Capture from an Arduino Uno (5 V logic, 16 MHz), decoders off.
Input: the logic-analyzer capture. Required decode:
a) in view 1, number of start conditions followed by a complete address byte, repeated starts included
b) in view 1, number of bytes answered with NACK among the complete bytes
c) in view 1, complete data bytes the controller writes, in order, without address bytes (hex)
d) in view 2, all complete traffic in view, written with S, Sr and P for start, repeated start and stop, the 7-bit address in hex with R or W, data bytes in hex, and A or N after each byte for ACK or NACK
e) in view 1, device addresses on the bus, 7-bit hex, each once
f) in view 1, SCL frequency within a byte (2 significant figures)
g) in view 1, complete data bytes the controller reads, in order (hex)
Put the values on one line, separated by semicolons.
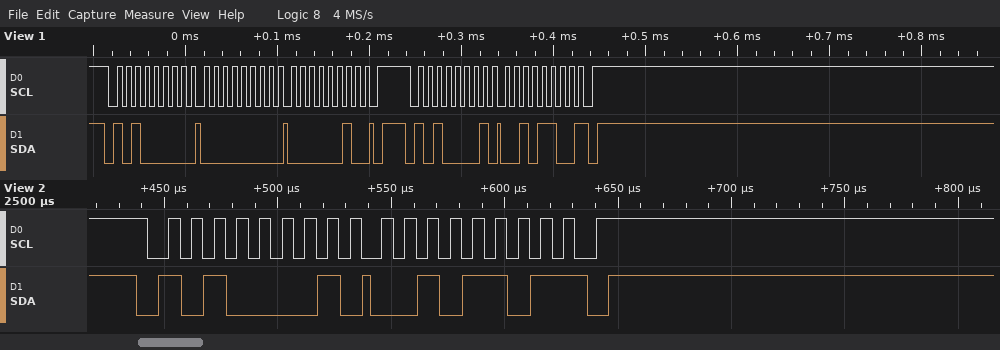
2; 1; 00 02; S 50R A 2D N P; 0x50; 100 kHz; 2C
